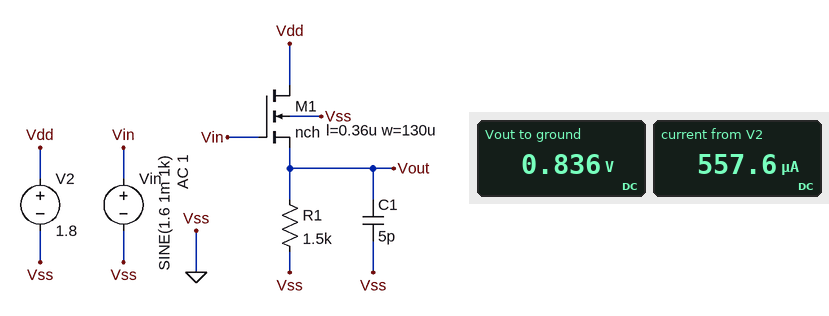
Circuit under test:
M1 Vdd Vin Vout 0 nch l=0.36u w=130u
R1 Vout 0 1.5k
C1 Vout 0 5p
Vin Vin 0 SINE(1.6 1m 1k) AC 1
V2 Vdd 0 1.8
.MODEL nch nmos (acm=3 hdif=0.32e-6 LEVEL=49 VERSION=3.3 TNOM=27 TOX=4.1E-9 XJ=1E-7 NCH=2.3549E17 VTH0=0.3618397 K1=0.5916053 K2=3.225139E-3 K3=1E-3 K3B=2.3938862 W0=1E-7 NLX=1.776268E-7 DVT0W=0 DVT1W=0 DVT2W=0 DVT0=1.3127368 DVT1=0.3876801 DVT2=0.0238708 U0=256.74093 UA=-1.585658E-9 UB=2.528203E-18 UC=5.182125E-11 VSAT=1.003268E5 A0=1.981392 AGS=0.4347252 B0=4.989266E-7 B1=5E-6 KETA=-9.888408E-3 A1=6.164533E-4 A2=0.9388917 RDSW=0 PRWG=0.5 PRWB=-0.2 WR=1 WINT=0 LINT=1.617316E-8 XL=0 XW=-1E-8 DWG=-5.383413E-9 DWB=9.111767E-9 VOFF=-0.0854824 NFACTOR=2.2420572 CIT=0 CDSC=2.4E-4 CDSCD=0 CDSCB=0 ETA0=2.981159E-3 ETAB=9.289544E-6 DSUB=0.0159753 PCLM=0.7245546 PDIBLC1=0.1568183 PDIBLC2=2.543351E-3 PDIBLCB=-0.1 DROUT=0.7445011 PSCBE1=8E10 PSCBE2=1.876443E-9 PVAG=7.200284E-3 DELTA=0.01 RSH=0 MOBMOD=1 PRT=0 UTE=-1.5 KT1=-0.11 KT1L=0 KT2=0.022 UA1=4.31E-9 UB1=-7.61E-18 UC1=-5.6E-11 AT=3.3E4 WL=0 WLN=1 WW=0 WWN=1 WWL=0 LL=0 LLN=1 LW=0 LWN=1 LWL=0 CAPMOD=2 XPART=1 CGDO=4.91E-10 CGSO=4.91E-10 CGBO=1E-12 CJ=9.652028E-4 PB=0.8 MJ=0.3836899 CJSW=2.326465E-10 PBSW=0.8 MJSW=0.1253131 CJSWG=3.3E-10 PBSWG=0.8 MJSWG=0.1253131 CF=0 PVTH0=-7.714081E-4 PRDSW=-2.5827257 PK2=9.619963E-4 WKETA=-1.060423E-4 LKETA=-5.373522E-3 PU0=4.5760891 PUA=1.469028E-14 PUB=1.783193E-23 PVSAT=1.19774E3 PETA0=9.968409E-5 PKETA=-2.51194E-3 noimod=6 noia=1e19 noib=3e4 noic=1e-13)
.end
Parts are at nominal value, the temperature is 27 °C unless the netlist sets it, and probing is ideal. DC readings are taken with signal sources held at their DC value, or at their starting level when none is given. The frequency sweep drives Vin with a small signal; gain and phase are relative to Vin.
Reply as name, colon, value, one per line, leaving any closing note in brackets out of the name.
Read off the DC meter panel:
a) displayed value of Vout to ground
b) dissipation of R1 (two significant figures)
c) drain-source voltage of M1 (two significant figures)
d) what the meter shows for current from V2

displayed value of Vout to ground: 0.836 V
dissipation of R1: 470 µW
drain-source voltage of M1: 960 mV
what the meter shows for current from V2: 557.6 µA
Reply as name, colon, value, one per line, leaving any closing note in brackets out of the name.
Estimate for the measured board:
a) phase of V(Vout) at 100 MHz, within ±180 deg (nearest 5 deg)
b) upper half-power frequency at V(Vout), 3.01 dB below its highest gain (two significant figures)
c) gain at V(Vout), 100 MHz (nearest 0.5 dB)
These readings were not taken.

phase of V(Vout) at 100 MHz, within ±180 deg: -15 deg
upper half-power frequency at V(Vout), 3.01 dB below its highest gain: 350 MHz
gain at V(Vout), 100 MHz: -2.5 dB
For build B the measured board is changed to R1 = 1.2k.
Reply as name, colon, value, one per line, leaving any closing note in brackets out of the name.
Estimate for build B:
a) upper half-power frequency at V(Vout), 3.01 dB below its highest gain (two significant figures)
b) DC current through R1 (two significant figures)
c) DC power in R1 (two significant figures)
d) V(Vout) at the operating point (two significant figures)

upper half-power frequency at V(Vout), 3.01 dB below its highest gain: 400 MHz
DC current through R1: 690 µA
DC power in R1: 570 µW
V(Vout) at the operating point: 830 mV
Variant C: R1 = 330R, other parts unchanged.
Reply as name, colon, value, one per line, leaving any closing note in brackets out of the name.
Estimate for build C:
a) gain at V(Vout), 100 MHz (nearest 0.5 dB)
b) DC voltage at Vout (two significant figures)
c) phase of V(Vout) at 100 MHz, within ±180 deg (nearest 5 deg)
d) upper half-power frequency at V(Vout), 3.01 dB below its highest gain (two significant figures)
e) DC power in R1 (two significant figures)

gain at V(Vout), 100 MHz: -3.0 dB
DC voltage at Vout: 740 mV
phase of V(Vout) at 100 MHz, within ±180 deg: -5 deg
upper half-power frequency at V(Vout), 3.01 dB below its highest gain: 810 MHz
DC power in R1: 1.7 mW
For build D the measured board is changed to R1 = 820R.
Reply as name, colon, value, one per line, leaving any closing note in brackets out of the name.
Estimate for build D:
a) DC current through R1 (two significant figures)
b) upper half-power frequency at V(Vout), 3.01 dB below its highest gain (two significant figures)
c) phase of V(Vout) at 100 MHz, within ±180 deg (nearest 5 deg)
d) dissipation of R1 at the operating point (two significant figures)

DC current through R1: 980 µA
upper half-power frequency at V(Vout), 3.01 dB below its highest gain: 510 MHz
phase of V(Vout) at 100 MHz, within ±180 deg: -10 deg
dissipation of R1 at the operating point: 790 µW
